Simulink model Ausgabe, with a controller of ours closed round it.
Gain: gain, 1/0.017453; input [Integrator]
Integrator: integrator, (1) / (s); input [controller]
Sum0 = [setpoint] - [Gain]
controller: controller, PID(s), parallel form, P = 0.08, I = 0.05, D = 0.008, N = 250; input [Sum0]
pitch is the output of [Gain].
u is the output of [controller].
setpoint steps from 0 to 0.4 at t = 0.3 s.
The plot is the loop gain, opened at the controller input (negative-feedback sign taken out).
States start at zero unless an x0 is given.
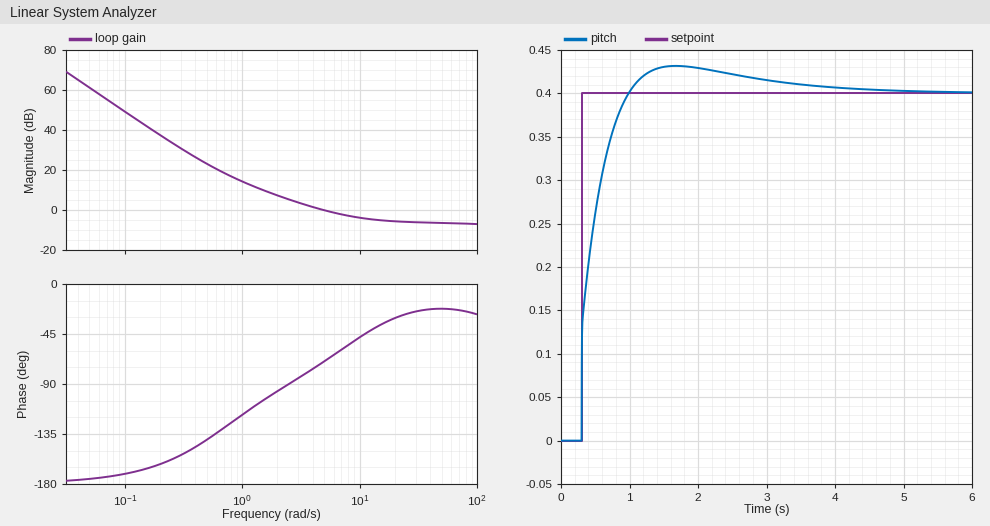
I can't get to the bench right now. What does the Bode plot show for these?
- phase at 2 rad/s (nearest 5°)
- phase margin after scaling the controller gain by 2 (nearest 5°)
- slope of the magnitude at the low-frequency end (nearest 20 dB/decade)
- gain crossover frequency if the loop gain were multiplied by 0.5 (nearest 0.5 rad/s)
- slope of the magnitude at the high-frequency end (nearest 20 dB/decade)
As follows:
-95°
155°
-40 dB/decade
2.5 rad/s
0 dB/decade
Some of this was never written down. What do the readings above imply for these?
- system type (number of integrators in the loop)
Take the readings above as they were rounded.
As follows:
2
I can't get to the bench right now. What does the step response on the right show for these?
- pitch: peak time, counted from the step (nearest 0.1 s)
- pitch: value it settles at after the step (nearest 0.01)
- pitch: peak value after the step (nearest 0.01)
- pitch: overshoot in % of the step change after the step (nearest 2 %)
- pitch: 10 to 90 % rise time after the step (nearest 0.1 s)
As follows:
1.4 s
0.40
0.43
8 %
0.5 s
